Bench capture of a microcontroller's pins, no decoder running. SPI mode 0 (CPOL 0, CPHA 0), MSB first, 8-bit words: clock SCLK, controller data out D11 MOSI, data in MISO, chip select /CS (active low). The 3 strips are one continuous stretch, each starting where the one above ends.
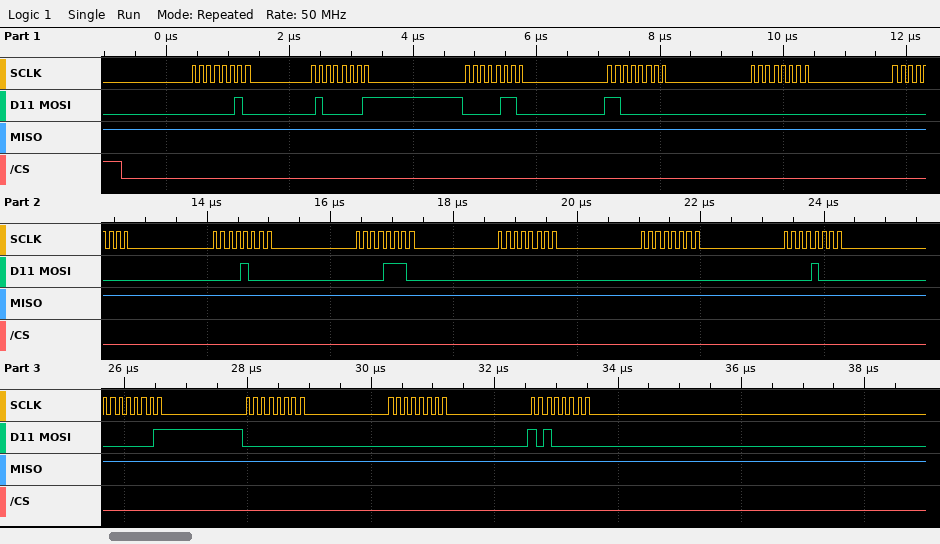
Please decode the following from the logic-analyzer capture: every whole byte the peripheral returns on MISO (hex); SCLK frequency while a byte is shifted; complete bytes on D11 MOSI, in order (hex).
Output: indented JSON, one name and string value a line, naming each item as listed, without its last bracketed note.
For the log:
{
  "every whole byte the peripheral returns on MISO": "FF FF FF FF FF FF FF FF FF FF FF FF FF FF FF",
  "SCLK frequency while a byte is shifted": "8 MHz",
  "complete bytes on D11 MOSI, in order": "02 41 06 C0 00 00 08 0E 00 00 08 01 00 00 A0"
}
